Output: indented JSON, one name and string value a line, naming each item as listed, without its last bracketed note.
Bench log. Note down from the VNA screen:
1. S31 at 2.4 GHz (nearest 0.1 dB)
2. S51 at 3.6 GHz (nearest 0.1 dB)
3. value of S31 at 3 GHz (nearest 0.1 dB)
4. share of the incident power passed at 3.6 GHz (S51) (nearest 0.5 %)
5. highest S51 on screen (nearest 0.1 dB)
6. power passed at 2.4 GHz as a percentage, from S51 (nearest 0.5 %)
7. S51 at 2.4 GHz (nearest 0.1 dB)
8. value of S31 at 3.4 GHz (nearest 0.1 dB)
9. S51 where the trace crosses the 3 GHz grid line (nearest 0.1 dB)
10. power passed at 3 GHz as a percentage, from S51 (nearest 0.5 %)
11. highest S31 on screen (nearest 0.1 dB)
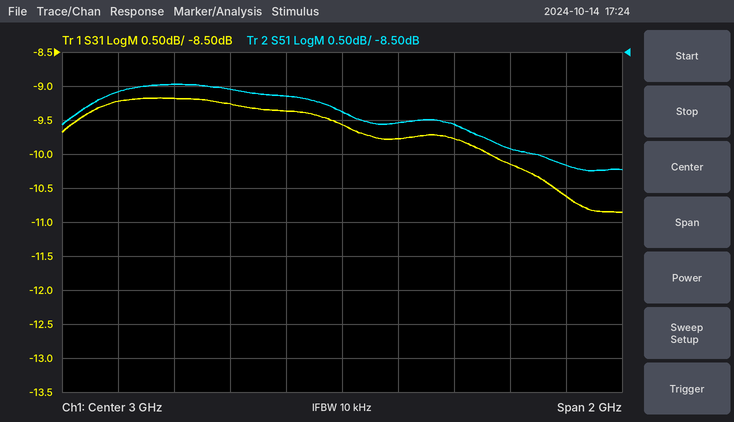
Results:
{
  "S31 at 2.4 GHz": "-9.2 dB",
  "S51 at 3.6 GHz": "-9.9 dB",
  "value of S31 at 3 GHz": "-9.6 dB",
  "share of the incident power passed at 3.6 GHz (S51)": "10.0 %",
  "highest S51 on screen": "-9.0 dB",
  "power passed at 2.4 GHz as a percentage, from S51": "12.5 %",
  "S51 at 2.4 GHz": "-9.0 dB",
  "value of S31 at 3.4 GHz": "-9.8 dB",
  "S51 where the trace crosses the 3 GHz grid line": "-9.4 dB",
  "power passed at 3 GHz as a percentage, from S51": "11.5 %",
  "highest S31 on screen": "-9.2 dB"
}
